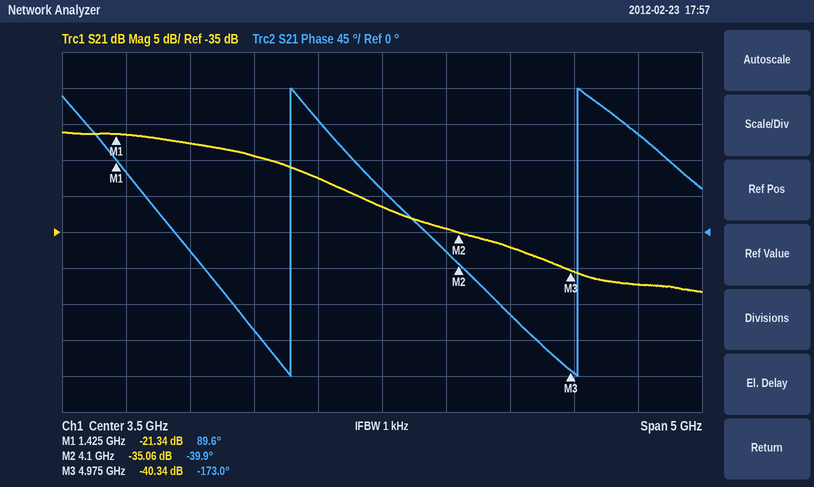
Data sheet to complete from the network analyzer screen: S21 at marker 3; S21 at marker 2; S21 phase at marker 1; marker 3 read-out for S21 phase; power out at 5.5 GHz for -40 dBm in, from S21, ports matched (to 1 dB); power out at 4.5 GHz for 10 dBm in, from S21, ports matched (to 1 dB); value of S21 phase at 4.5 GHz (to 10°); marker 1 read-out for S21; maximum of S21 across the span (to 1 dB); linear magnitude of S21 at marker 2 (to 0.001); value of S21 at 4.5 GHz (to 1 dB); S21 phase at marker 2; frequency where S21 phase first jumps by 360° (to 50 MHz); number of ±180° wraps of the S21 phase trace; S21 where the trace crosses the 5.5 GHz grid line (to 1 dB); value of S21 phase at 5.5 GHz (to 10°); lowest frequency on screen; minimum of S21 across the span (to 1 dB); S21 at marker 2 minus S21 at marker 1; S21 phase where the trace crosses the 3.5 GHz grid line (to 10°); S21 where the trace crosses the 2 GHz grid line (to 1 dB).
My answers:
-40.34 dB
-35.06 dB
89.6°
-173.0°
-82 dBm
-27 dBm
-100°
-21.34 dB
-21 dB
0.018
-37 dB
-39.9°
2.80 GHz
2
-42 dB
120°
1 GHz
-43 dB
-13.72 dB
50°
-23 dB
